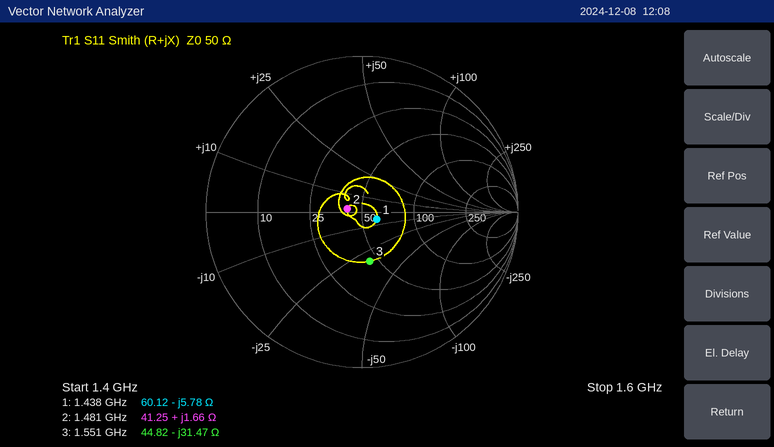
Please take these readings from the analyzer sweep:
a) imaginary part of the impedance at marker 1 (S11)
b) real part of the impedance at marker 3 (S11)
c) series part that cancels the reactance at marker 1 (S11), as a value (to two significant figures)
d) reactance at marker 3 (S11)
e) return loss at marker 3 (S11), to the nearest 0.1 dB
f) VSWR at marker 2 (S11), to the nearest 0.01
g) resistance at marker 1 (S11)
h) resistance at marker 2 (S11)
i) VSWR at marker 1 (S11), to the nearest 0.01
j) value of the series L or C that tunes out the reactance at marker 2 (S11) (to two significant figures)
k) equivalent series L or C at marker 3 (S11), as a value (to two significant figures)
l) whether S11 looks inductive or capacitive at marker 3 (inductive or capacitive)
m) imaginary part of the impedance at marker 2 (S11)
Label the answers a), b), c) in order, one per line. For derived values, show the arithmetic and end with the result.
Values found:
a) -5.78 Ω
b) 44.82 Ω
c) L = 5.78 Ω/(2π × 1.438 GHz) ≈ 640 pH
d) -31.47 Ω
e) 9.9 dB
f) 1.22
g) 60.12 Ω
h) 41.25 Ω
i) 1.24
j) C = 1/(2π × 1.481 GHz × 1.66 Ω) ≈ 65 pF
k) C = 1/(2π × 1.551 GHz × 31.47 Ω) ≈ 3.3 pF
l) capacitive
m) +1.66 Ω
